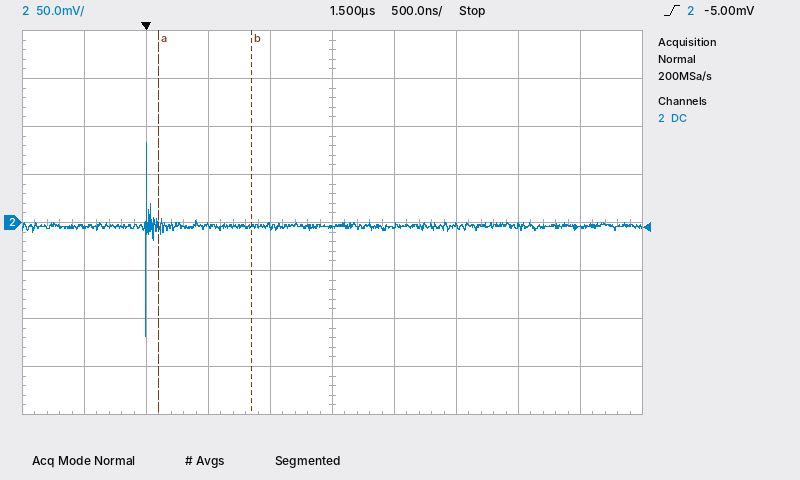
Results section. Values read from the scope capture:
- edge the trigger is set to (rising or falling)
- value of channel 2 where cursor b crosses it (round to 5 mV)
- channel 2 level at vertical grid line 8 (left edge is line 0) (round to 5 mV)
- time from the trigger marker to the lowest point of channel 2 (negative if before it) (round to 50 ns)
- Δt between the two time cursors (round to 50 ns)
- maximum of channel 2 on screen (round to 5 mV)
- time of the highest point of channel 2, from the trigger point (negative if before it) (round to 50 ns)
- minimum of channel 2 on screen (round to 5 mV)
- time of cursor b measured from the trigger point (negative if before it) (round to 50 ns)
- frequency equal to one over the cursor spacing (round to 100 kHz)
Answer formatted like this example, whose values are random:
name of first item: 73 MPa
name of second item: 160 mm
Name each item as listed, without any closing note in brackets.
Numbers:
edge the trigger is set to: rising
value of channel 2 where cursor b crosses it: -5 mV
channel 2 level at vertical grid line 8 (left edge is line 0): -5 mV
time from the trigger marker to the lowest point of channel 2 (negative if before it): 0 ns
Δt between the two time cursors: 750 ns
maximum of channel 2 on screen: 85 mV
time of the highest point of channel 2, from the trigger point (negative if before it): 0 ns
minimum of channel 2 on screen: -120 mV
time of cursor b measured from the trigger point (negative if before it): +850 ns
frequency equal to one over the cursor spacing: 1.3 MHz
